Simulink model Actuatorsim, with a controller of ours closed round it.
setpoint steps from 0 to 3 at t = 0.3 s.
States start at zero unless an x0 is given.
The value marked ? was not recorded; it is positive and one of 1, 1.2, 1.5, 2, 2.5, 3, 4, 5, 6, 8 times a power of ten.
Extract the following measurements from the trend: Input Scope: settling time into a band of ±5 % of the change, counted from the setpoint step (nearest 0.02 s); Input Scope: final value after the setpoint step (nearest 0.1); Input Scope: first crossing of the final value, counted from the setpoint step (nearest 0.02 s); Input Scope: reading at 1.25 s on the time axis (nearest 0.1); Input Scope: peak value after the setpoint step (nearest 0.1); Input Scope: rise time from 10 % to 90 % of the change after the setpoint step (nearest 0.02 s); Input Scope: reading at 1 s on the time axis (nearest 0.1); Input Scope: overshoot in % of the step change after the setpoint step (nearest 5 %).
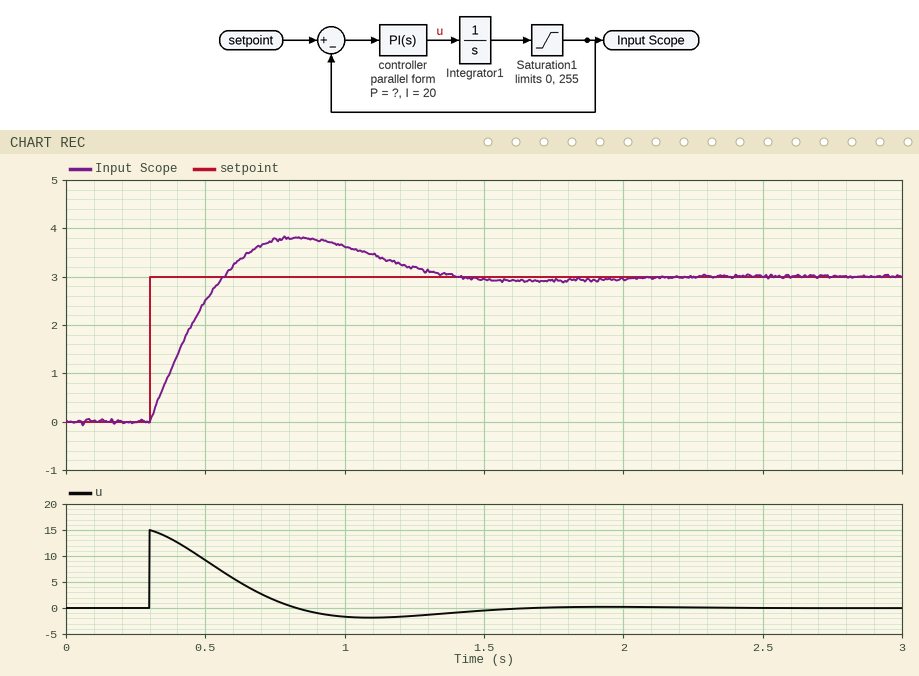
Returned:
0.98 s
3.0
0.26 s
3.2
3.8
0.20 s
3.6
25 %
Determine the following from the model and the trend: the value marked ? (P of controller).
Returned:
5
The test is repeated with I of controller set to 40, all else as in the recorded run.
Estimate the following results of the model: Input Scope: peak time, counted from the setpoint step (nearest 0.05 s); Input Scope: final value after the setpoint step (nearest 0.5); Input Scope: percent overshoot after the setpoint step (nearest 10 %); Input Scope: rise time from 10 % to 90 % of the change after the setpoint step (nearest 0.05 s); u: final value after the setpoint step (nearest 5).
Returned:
0.40 s
3.0
40 %
0.15 s
0
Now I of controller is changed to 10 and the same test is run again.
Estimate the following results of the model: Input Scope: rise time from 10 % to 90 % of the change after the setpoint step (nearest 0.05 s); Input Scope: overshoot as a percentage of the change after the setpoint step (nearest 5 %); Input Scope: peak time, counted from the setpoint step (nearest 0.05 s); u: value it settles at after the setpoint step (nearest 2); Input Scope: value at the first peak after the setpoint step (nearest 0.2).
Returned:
0.25 s
20 %
0.70 s
0
3.6
